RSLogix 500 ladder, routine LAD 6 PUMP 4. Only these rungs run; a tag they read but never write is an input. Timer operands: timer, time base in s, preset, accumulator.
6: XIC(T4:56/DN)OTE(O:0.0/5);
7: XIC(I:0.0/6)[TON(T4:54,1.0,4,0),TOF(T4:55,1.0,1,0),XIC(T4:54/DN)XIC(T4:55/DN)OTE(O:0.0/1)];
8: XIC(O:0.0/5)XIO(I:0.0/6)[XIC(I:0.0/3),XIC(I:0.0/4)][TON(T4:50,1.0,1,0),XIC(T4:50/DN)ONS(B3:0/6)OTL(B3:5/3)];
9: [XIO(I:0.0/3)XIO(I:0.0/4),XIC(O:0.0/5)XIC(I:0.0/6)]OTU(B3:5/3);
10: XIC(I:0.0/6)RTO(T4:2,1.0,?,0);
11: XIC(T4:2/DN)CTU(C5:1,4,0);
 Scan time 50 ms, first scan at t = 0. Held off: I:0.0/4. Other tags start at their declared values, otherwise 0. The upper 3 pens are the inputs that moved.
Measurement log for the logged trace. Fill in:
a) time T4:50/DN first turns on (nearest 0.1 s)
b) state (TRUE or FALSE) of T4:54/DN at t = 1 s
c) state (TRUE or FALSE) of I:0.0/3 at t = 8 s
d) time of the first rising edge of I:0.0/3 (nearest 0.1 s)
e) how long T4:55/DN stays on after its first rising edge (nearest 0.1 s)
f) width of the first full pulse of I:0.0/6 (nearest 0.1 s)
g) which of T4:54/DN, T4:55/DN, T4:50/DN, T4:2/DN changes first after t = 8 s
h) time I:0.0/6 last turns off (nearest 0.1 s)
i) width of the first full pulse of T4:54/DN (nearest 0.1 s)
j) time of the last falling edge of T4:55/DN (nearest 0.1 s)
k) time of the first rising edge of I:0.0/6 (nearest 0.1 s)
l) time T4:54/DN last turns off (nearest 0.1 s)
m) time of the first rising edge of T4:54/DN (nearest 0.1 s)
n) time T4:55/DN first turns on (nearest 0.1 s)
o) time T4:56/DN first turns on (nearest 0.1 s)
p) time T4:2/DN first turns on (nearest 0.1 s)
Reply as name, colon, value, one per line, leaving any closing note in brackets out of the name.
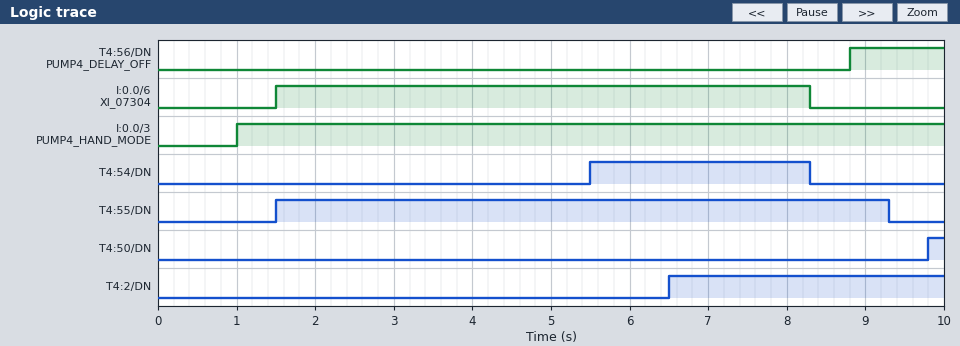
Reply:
time T4:50/DN first turns on: 9.8 s
state (TRUE or FALSE) of T4:54/DN at t = 1 s: FALSE
state (TRUE or FALSE) of I:0.0/3 at t = 8 s: TRUE
time of the first rising edge of I:0.0/3: 1.0 s
how long T4:55/DN stays on after its first rising edge: 7.8 s
width of the first full pulse of I:0.0/6: 6.8 s
which of T4:54/DN, T4:55/DN, T4:50/DN, T4:2/DN changes first after t = 8 s: T4:54/DN
time I:0.0/6 last turns off: 8.3 s
width of the first full pulse of T4:54/DN: 2.8 s
time of the last falling edge of T4:55/DN: 9.3 s
time of the first rising edge of I:0.0/6: 1.5 s
time T4:54/DN last turns off: 8.3 s
time of the first rising edge of T4:54/DN: 5.5 s
time T4:55/DN first turns on: 1.5 s
time T4:56/DN first turns on: 8.8 s
time T4:2/DN first turns on: 6.5 s
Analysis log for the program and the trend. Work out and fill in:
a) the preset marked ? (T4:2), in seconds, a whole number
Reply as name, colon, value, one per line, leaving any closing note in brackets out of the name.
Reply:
the preset marked ? (T4:2), in seconds, a whole number: 5 s
